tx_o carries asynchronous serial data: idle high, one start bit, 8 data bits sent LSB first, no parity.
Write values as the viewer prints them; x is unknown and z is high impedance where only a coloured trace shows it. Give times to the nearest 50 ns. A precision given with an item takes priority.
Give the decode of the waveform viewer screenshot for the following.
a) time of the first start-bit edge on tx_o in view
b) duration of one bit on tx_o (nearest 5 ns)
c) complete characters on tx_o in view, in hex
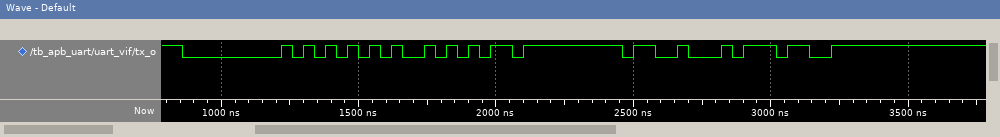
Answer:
850 ns
40 ns
00, 55, AA, FF, 13, 37
